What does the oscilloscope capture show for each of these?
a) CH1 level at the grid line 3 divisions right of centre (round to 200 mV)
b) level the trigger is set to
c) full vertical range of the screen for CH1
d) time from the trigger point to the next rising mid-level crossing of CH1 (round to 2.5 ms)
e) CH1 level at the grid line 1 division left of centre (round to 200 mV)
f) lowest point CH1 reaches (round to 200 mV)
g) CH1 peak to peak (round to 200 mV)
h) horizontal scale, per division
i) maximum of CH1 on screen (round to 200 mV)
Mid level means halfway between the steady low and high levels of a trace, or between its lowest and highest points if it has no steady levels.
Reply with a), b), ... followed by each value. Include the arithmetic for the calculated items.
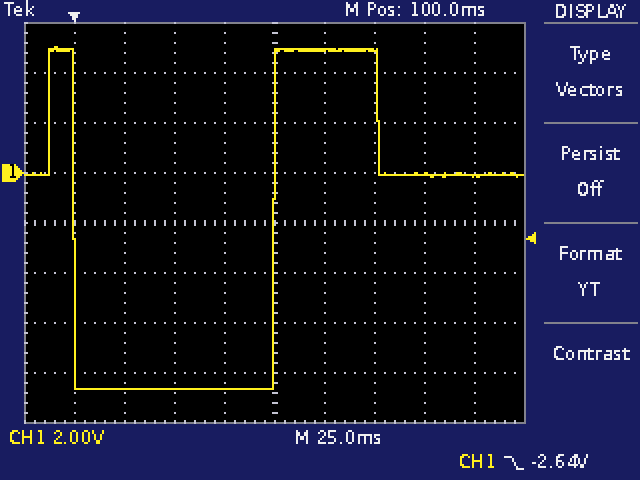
a) 0.0 V
b) -2.64 V
c) 16 V
d) 100.0 ms
e) -8.6 V
f) -8.6 V
g) 5.0 V − (-8.6 V) = 13.6 V
h) 25 ms
i) 5.0 V
